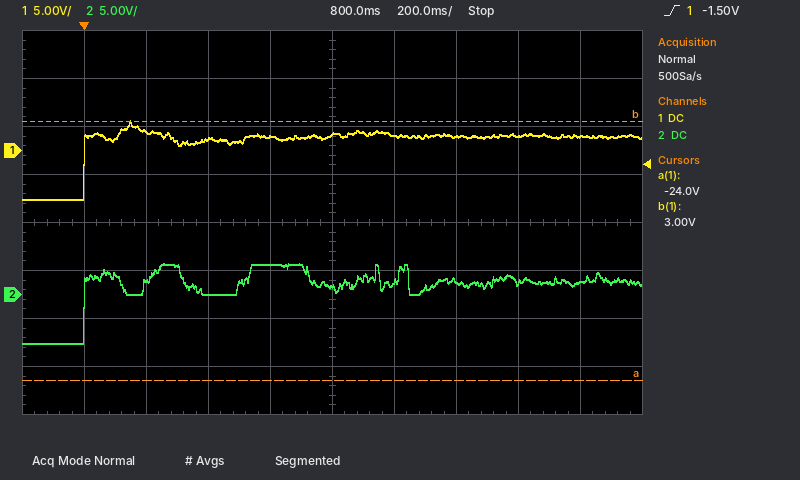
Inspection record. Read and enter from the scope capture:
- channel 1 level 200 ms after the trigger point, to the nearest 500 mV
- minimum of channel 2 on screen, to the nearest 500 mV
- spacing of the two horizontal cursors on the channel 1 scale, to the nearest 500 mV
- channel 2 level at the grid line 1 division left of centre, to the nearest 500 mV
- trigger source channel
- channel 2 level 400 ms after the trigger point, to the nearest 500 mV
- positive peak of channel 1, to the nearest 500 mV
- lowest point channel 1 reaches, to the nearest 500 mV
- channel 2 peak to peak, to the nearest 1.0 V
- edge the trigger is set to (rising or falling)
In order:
2.0 V
-5.0 V
27.0 V
3.0 V
channel 1
0.0 V
3.0 V
-5.0 V
8.0 V
rising
